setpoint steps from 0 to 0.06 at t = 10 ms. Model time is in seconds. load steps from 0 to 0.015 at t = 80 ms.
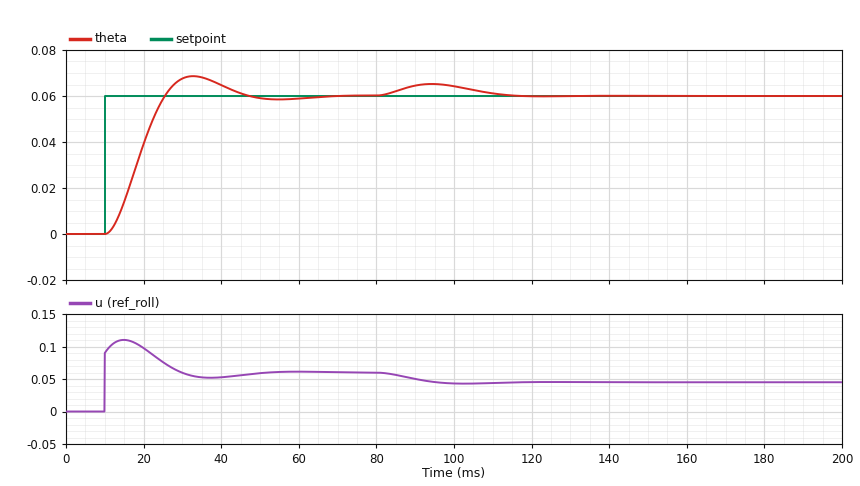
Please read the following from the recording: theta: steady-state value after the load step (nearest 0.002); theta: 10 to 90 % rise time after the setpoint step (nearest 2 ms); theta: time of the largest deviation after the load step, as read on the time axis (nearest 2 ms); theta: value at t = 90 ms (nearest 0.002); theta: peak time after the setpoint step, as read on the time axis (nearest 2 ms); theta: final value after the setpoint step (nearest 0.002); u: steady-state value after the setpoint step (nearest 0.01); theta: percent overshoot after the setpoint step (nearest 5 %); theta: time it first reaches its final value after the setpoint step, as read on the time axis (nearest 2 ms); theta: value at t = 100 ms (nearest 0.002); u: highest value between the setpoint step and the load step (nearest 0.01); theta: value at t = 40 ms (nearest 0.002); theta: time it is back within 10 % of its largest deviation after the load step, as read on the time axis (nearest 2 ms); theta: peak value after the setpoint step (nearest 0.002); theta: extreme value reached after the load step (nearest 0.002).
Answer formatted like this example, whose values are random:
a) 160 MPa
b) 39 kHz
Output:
a) 0.060
b) 10 ms
c) 94 ms
d) 0.064
e) 32 ms
f) 0.060
g) 0.06
h) 15 %
i) 26 ms
j) 0.064
k) 0.11
l) 0.064
m) 114 ms
n) 0.068
o) 0.066
